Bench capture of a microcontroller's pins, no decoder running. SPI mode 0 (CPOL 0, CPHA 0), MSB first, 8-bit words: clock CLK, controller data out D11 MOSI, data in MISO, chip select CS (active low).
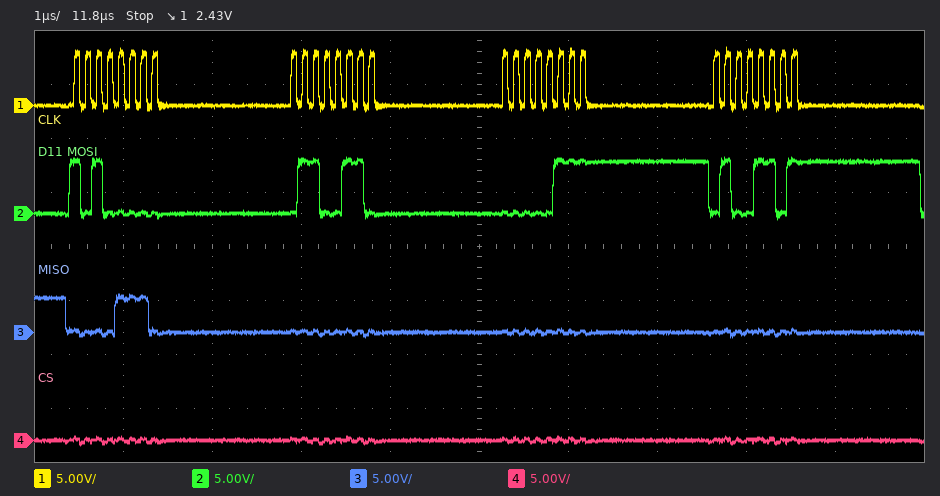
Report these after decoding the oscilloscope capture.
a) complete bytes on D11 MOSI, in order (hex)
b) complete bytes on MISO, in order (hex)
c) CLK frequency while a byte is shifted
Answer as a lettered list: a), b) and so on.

a) A0 66 07 4D
b) 0E 00 00 00
c) 8 MHz
